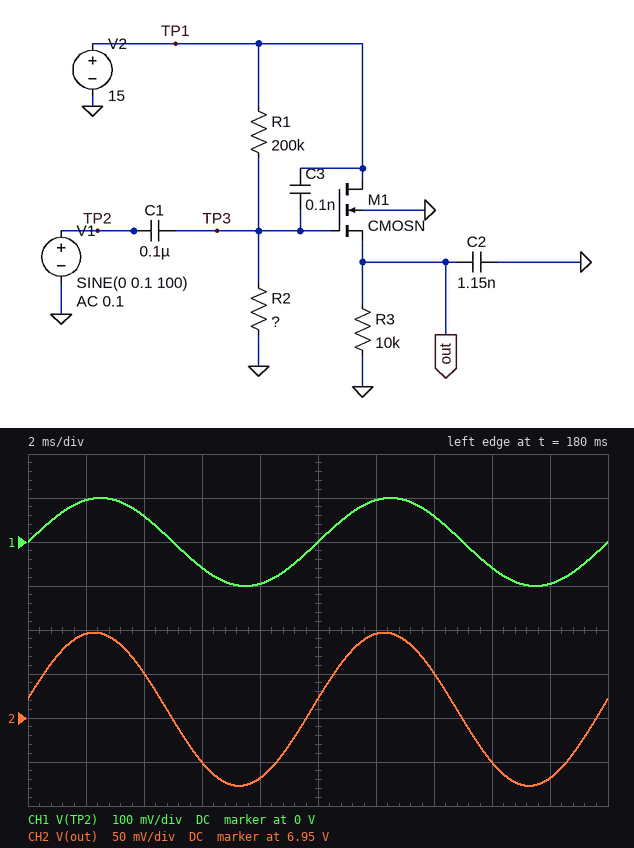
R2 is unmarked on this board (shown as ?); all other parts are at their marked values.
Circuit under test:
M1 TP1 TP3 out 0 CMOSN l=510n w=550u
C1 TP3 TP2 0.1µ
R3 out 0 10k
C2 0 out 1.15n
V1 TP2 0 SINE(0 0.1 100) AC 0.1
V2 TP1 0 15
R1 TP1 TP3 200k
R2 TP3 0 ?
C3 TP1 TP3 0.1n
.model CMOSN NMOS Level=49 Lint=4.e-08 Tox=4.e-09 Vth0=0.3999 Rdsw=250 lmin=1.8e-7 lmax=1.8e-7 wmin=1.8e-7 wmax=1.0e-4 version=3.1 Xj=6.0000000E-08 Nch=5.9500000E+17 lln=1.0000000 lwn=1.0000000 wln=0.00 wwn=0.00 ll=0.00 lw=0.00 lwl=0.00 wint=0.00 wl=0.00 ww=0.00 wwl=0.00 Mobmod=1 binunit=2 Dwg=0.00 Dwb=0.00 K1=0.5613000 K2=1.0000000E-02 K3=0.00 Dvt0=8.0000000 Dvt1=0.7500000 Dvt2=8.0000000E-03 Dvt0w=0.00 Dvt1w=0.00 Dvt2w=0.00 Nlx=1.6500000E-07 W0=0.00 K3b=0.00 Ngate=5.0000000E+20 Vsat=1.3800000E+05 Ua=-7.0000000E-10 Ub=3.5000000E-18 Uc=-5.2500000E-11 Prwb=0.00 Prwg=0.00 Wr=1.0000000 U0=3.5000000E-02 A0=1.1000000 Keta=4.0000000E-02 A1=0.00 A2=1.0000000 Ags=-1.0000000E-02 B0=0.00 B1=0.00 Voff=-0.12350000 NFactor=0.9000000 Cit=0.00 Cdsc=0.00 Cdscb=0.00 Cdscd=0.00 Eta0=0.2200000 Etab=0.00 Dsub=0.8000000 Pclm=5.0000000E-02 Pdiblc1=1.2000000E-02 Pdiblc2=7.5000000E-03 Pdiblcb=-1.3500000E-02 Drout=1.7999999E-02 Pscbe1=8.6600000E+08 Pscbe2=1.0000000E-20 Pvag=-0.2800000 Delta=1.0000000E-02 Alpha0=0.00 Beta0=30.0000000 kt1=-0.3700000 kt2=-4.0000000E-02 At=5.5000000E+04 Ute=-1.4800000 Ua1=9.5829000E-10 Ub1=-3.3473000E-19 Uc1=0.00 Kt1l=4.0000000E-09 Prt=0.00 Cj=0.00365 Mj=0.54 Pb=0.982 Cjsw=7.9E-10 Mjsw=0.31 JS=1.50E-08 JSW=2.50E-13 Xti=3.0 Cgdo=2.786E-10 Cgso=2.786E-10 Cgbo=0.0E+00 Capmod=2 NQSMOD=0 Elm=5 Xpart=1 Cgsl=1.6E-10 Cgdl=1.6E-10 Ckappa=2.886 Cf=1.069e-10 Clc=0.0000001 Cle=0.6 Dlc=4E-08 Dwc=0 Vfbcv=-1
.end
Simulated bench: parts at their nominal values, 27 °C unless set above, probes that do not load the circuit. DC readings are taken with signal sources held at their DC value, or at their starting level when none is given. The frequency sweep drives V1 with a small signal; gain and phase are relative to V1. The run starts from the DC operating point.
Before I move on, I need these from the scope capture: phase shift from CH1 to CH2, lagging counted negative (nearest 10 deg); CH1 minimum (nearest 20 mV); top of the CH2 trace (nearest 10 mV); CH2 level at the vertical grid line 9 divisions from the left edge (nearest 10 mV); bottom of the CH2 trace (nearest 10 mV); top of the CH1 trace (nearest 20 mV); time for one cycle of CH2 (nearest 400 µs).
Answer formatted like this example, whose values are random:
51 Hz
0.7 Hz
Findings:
10 deg
-100 mV
7.05 V
6.88 V
6.87 V
100 mV
10.0 ms
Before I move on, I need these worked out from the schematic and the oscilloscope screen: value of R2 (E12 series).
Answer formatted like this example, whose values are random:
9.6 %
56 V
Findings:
270 kΩ
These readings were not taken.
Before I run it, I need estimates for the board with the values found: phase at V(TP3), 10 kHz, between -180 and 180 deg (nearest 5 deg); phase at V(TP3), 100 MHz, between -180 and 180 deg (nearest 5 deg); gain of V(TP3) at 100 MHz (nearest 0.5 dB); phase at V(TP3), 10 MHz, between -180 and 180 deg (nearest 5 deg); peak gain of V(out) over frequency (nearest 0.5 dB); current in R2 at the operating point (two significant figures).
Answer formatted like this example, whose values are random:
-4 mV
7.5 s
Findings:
0 deg
0 deg
0 dB
0 deg
-1.0 dB
32 µA
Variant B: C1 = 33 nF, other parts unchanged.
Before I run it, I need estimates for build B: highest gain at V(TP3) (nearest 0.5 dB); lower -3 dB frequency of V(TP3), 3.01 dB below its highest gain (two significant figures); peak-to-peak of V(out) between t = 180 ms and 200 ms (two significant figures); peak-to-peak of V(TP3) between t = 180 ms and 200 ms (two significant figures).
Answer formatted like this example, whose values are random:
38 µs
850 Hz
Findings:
0 dB
42 Hz
160 mV
180 mV
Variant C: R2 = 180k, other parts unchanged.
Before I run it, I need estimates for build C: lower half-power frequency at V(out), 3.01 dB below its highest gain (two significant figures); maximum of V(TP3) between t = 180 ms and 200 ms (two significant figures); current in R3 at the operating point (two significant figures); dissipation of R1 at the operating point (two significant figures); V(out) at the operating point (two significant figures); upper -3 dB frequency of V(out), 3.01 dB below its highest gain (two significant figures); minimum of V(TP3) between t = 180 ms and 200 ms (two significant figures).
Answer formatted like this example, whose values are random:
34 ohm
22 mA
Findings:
17 Hz
7.2 V
560 µA
310 µW
5.6 V
1.6 MHz
7.0 V
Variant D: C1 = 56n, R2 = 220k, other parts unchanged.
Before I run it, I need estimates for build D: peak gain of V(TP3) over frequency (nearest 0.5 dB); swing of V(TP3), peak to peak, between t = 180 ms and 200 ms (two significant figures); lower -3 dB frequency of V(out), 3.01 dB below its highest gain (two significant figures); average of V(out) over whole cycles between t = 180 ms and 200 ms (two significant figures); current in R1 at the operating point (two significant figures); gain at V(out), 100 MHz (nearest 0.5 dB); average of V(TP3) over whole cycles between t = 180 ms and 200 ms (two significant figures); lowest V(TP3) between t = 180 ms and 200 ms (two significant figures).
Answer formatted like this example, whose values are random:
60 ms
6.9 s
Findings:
0 dB
190 mV
27 Hz
6.3 V
36 µA
-37.0 dB
7.9 V
7.8 V
